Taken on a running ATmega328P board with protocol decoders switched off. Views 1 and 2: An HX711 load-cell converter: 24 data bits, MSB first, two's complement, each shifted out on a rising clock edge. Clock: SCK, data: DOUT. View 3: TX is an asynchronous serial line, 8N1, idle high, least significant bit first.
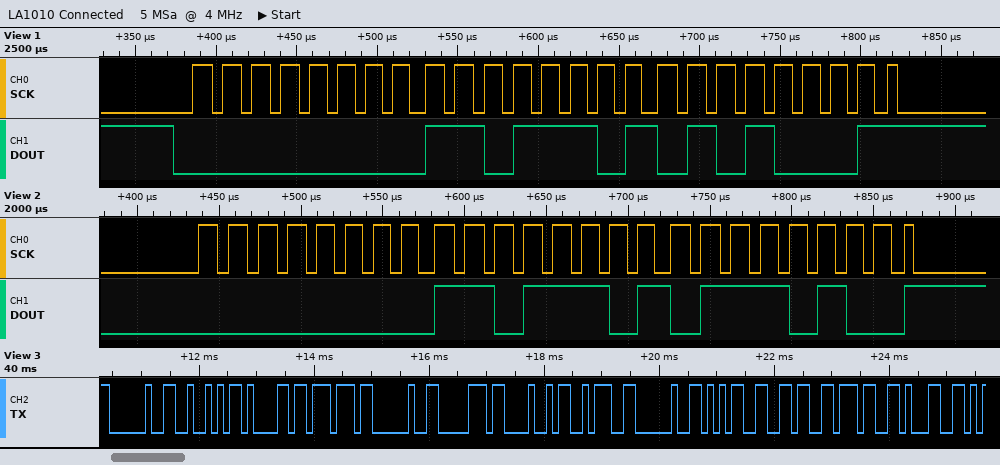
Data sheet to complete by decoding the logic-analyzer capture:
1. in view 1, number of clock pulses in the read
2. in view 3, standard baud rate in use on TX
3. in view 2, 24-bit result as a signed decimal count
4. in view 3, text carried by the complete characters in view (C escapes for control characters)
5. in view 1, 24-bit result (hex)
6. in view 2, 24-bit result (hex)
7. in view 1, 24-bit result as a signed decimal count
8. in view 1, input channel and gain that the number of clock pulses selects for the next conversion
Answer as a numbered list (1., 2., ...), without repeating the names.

1. 25
2. 9600 baud
3. 56692
4. " Raw pH: 5671"
5. 0x00DD51
6. 0x00DD74
7. 56657
8. channel A, gain 128
